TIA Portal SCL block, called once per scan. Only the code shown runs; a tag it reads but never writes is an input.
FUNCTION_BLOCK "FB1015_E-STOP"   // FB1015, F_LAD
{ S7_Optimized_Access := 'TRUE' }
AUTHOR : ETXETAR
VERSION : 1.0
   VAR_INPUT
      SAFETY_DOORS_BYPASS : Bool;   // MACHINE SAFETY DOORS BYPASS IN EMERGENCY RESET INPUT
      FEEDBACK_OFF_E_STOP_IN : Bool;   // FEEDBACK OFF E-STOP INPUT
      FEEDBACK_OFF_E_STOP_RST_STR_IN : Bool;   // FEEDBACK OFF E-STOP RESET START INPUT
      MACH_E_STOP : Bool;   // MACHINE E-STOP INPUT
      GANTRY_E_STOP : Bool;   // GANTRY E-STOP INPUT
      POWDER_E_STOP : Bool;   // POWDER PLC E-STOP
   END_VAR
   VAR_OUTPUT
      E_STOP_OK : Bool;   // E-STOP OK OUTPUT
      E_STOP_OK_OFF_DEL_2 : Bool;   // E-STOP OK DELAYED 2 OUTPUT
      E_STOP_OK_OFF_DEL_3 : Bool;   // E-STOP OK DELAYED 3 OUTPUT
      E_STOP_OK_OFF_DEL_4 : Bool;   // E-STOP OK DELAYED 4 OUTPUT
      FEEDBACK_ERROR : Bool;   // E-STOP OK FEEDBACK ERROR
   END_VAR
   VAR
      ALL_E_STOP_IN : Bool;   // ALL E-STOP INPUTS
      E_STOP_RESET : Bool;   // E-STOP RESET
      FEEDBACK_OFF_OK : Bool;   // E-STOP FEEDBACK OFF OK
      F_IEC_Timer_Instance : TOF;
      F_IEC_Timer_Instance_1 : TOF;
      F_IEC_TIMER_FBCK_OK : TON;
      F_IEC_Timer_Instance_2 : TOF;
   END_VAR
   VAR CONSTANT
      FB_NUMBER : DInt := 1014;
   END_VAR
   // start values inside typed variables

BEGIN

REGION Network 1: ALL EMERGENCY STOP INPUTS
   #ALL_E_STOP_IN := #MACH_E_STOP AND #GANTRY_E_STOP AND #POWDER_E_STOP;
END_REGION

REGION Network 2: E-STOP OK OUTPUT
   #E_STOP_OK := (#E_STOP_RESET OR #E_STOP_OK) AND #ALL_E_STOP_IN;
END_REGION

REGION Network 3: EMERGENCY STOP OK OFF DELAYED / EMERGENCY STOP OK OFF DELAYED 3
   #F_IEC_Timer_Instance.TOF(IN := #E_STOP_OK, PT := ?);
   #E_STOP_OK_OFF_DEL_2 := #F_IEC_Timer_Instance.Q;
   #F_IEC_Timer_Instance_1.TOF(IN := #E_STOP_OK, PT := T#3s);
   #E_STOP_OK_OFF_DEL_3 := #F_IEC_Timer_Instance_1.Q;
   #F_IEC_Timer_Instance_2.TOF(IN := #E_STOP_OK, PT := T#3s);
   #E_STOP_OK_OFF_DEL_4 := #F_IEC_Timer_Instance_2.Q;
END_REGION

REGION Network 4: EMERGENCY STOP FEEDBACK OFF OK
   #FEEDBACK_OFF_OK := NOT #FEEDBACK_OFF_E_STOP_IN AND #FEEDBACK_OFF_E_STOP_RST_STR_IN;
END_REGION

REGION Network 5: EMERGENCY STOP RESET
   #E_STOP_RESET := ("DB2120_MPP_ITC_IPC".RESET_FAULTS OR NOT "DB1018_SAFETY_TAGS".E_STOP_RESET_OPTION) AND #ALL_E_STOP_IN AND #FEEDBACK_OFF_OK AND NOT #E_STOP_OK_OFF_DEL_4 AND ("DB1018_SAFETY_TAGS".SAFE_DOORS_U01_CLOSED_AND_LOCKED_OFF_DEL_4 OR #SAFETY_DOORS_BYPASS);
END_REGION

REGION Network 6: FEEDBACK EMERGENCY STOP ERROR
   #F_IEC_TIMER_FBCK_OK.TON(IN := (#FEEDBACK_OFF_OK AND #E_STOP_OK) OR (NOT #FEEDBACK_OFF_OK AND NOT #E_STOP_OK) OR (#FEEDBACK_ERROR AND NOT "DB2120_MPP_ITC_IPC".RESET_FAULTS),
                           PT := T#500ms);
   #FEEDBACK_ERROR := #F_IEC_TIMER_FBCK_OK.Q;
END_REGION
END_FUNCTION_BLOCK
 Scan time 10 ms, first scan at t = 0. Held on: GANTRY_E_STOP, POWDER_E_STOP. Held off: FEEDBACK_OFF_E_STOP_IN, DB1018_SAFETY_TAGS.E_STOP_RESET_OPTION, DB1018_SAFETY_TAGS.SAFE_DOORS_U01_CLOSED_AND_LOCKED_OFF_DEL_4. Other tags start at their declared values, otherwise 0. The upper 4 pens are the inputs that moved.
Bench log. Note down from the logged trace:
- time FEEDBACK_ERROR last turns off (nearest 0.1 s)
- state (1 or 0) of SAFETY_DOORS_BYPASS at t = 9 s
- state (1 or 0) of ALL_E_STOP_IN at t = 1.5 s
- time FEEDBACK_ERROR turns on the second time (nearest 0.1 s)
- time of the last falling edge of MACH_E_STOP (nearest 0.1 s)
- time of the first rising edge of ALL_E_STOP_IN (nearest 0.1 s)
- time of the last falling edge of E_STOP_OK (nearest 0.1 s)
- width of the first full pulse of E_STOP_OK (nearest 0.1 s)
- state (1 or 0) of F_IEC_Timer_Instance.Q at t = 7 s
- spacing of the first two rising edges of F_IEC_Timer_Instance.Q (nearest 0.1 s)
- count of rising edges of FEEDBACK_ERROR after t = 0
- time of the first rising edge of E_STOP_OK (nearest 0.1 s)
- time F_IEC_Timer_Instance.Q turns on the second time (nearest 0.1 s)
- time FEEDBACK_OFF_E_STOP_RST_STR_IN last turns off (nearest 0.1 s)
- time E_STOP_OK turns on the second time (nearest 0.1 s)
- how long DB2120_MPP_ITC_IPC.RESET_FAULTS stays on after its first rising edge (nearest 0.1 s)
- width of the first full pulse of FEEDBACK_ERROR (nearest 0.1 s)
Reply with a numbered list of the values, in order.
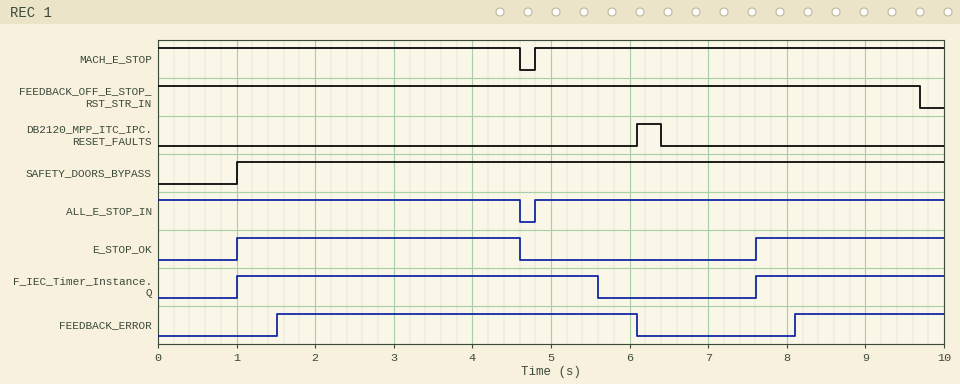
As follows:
1. 6.1 s
2. 1
3. 1
4. 8.1 s
5. 4.6 s
6. 4.8 s
7. 4.6 s
8. 3.6 s
9. 0
10. 6.6 s
11. 2
12. 1.0 s
13. 7.6 s
14. 9.7 s
15. 7.6 s
16. 0.3 s
17. 4.6 s
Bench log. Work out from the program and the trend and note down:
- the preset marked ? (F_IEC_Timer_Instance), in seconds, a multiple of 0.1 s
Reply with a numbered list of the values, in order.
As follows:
1. 1.0 s
